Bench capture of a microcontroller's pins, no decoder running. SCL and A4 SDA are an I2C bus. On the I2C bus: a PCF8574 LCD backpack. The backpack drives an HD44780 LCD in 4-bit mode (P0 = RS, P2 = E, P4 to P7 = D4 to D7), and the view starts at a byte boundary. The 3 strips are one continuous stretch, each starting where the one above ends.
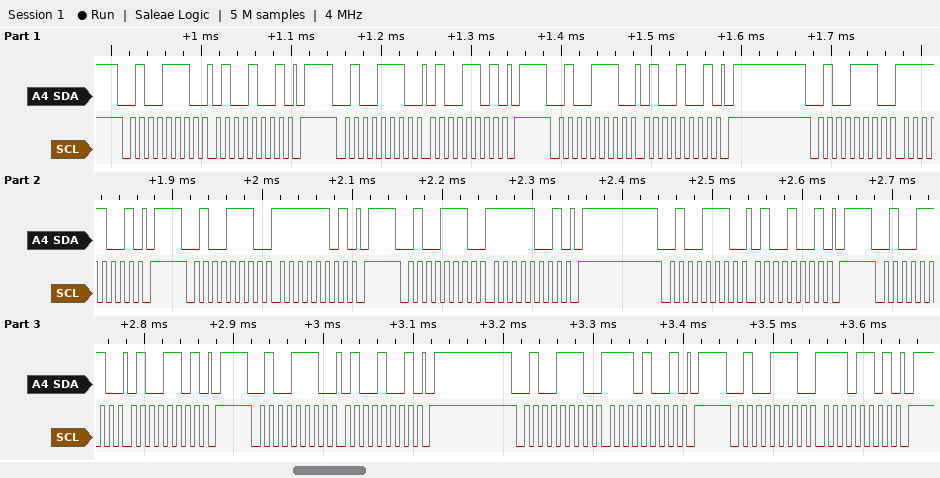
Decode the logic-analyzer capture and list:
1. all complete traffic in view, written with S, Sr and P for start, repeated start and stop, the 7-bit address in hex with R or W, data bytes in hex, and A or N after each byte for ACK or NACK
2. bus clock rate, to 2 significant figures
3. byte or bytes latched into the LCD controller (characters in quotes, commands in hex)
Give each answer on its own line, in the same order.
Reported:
S 27W A 49 A P S 27W A 4D A P S 27W A 49 A P S 27W A F9 A P S 27W A FD A P S 27W A F9 A P S 27W A 49 A P S 27W A 4D A P S 27W A 49 A P S 27W A E9 A P S 27W A ED A P
100 kHz
'O'
